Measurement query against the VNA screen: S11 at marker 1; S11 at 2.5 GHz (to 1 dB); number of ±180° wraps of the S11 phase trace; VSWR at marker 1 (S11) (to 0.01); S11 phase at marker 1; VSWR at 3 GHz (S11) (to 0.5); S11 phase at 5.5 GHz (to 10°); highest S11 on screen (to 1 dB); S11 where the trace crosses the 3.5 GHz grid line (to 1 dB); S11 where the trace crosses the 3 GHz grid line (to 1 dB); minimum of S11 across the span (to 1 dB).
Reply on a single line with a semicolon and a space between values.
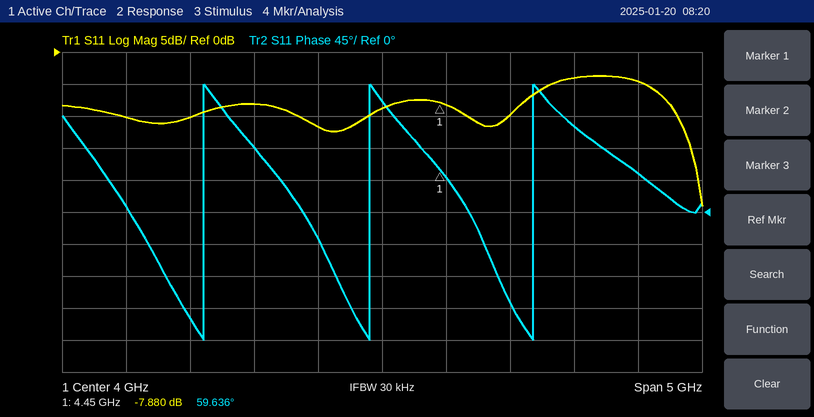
-7.880 dB; -10 dB; 3; 2.35; 59.636°; 2.5; 120°; -4 dB; -12 dB; -8 dB; -24 dB
